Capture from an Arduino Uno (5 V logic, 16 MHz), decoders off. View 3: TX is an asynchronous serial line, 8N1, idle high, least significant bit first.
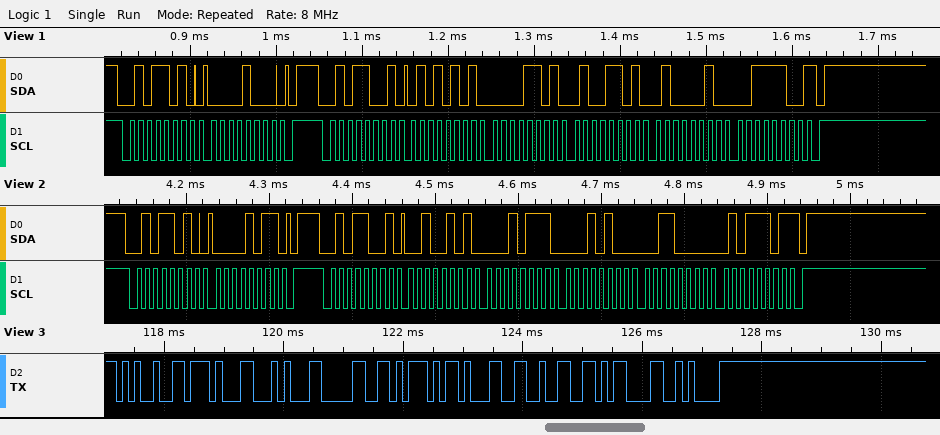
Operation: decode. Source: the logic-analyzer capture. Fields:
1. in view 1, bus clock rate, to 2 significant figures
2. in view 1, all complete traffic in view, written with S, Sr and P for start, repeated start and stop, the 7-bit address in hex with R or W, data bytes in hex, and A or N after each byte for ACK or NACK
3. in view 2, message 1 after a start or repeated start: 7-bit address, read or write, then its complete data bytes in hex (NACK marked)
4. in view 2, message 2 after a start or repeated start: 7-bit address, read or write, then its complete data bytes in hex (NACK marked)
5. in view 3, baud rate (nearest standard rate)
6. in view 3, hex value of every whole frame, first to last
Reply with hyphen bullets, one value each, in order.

- 100 kHz
- S 2DW A 08 A P S 2CR A 55 A 0D A 4D A 42 A 3C N P
- 0x2D write: 0B
- 0x2C read: 25 17 14 30 5D NACK
- 9600 baud
- 25 17 14 30 5D 31 32 0D 0A
